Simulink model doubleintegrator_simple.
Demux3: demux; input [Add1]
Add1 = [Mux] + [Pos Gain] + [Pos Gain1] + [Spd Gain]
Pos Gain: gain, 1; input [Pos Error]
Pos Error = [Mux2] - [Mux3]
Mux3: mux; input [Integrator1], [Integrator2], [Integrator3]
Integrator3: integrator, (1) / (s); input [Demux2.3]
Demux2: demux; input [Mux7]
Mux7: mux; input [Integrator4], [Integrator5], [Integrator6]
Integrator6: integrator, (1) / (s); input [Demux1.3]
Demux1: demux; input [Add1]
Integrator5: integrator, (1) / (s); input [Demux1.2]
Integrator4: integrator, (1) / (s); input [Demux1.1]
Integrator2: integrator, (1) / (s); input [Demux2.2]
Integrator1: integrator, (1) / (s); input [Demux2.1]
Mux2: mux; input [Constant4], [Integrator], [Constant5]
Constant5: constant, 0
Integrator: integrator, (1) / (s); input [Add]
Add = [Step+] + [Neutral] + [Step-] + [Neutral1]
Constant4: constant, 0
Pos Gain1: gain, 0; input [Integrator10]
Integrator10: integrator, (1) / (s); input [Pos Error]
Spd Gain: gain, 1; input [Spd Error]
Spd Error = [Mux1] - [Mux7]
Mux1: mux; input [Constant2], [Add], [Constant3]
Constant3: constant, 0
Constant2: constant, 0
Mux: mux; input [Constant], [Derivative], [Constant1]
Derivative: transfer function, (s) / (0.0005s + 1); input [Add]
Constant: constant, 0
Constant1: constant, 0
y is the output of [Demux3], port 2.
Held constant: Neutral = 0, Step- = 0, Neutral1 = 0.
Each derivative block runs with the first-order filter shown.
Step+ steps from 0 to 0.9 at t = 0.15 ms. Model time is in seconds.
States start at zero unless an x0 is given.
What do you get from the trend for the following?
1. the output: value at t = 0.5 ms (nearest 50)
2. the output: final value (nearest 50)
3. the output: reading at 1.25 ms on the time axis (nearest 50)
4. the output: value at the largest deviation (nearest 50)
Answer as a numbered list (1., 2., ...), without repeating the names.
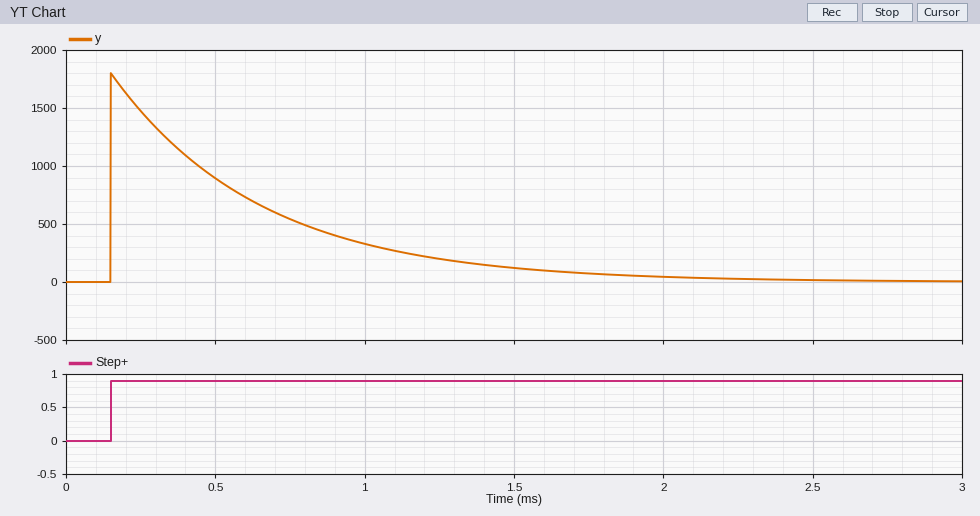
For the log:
1. 900
2. 0
3. 200
4. 1800
